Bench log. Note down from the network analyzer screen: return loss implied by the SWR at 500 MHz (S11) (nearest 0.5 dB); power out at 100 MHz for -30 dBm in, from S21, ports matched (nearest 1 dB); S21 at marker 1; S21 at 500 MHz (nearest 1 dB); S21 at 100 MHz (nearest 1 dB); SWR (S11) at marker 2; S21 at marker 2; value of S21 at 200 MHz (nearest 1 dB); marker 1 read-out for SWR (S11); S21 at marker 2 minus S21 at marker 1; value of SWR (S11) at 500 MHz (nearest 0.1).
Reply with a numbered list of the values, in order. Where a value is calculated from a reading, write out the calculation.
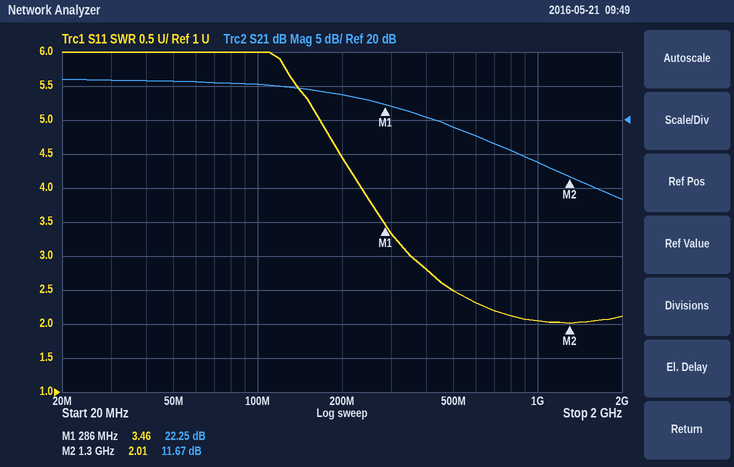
1. −20 log10((2.5 − 1)/(2.5 + 1)) ≈ 7.36 dB, so 7.5 dB to the nearest 0.5 dB
2. -30 dBm + (25 dB) = -5 dBm
3. 22.25 dB
4. 19 dB
5. 25 dB
6. 2.01
7. 11.67 dB
8. 24 dB
9. 3.46
10. 11.67 − (22.25) = -10.58 dB
11. 2.5
